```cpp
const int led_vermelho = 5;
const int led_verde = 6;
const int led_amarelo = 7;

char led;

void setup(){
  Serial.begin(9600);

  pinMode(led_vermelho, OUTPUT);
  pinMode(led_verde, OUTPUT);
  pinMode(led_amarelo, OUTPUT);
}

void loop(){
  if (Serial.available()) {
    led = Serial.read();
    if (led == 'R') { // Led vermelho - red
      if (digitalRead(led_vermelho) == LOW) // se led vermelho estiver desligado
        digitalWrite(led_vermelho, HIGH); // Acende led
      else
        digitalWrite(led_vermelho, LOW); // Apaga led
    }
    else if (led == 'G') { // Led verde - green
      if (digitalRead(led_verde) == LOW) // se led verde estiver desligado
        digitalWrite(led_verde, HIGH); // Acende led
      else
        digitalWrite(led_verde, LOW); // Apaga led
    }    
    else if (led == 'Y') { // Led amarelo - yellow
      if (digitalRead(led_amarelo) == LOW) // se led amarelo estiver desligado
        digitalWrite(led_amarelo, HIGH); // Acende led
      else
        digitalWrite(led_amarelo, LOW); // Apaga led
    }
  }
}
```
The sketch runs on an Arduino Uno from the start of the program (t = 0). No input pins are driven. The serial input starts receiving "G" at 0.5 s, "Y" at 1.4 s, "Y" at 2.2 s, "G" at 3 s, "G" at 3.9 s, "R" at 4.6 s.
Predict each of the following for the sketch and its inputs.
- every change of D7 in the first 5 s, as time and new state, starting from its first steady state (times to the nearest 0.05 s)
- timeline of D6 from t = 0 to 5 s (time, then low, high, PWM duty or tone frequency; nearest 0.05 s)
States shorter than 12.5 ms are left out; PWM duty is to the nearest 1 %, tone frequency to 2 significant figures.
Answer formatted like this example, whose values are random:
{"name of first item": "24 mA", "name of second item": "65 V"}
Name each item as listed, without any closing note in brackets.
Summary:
{"every change of D7 in the first 5 s, as time and new state, starting from its first steady state": "0 s low; 1.4 s high; 2.2 s low", "timeline of D6 from t = 0 to 5 s": "0 s low; 0.5 s high; 3 s low; 3.9 s high"}
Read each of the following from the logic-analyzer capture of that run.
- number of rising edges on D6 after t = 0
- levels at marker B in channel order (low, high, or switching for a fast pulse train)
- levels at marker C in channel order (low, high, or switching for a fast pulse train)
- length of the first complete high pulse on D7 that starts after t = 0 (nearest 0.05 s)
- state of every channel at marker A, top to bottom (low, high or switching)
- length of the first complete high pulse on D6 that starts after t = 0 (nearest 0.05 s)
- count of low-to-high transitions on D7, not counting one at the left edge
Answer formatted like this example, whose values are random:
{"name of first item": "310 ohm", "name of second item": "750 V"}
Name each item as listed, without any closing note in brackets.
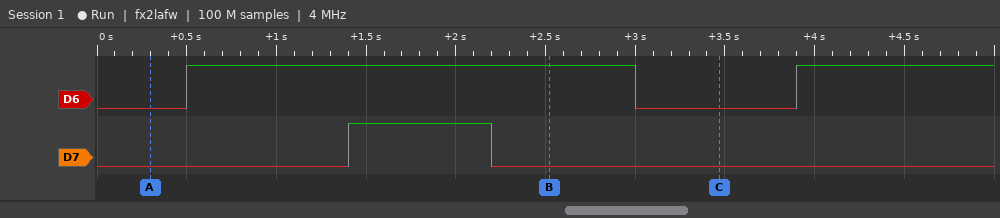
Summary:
{"number of rising edges on D6 after t = 0": "2", "levels at marker B in channel order": "D6 high, D7 low", "levels at marker C in channel order": "D6 low, D7 low", "length of the first complete high pulse on D7 that starts after t = 0": "0.80 s", "state of every channel at marker A, top to bottom": "D6 low, D7 low", "length of the first complete high pulse on D6 that starts after t = 0": "2.50 s", "count of low-to-high transitions on D7, not counting one at the left edge": "1"}
